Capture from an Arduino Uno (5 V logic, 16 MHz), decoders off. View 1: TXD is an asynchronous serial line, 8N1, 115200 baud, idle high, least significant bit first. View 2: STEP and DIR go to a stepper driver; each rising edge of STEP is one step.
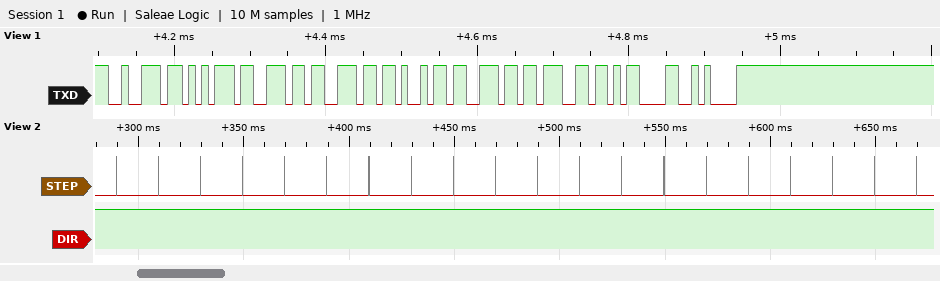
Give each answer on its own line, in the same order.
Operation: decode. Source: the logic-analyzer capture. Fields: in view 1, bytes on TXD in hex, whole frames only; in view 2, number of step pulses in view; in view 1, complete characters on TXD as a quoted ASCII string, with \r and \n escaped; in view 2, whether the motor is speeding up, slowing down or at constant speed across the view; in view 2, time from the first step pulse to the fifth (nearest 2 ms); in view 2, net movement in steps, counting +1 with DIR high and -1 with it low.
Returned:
72 75 6E 6E 69 6E 67 0D 0A
20
"running\r\n"
constant speed
80 ms
+20
